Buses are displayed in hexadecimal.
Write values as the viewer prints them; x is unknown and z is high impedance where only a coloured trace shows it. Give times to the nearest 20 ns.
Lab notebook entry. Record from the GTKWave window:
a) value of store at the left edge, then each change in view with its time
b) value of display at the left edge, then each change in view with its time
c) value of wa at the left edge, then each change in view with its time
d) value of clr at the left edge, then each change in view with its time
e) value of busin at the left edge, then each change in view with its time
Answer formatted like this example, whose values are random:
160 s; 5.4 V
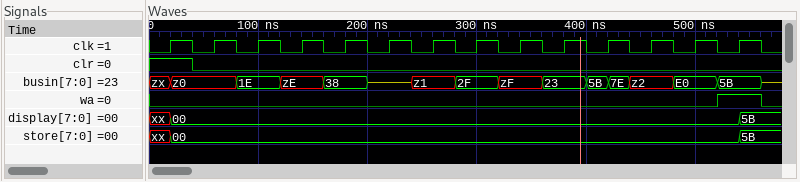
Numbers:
xx, 00 at 20 ns, 5B at 540 ns; xx, 00 at 20 ns, 5B at 540 ns; 0, 1 at 520 ns, 0 at 560 ns; 1, 0 at 40 ns; zx, z0 at 20 ns, 1E at 80 ns, zE at 120 ns, 38 at 160 ns, z at 200 ns, z1 at 240 ns, 2F at 280 ns, zF at 320 ns, 23 at 360 ns, 5B at 400 ns, 7E at 420 ns, z2 at 440 ns, E0 at 480 ns, 5B at 520 ns, z at 560 ns
